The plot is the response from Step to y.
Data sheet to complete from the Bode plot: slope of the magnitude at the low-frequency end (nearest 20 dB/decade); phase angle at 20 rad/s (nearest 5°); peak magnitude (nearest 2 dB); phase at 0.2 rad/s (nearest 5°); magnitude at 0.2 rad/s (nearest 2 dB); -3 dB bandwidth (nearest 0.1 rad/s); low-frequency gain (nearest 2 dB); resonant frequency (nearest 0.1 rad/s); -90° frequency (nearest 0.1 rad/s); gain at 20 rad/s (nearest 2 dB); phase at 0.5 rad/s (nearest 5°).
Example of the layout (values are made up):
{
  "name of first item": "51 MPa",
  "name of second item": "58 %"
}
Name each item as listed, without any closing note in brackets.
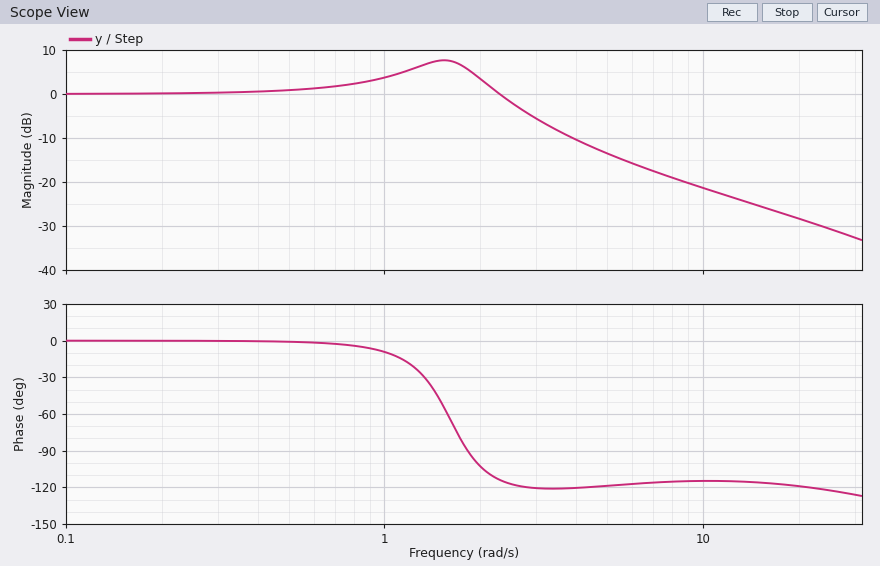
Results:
{
  "slope of the magnitude at the low-frequency end": "0 dB/decade",
  "phase angle at 20 rad/s": "-120°",
  "peak magnitude": "8 dB",
  "phase at 0.2 rad/s": "0°",
  "magnitude at 0.2 rad/s": "0 dB",
  "-3 dB bandwidth": "2.6 rad/s",
  "low-frequency gain": "0 dB",
  "resonant frequency": "1.5 rad/s",
  "-90° frequency": "1.8 rad/s",
  "gain at 20 rad/s": "-28 dB",
  "phase at 0.5 rad/s": "0°"
}
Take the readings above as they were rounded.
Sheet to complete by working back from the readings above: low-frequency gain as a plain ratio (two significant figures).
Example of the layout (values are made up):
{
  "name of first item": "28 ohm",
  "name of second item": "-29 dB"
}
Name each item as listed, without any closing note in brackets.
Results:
{
  "low-frequency gain as a plain ratio": "1.0"
}
